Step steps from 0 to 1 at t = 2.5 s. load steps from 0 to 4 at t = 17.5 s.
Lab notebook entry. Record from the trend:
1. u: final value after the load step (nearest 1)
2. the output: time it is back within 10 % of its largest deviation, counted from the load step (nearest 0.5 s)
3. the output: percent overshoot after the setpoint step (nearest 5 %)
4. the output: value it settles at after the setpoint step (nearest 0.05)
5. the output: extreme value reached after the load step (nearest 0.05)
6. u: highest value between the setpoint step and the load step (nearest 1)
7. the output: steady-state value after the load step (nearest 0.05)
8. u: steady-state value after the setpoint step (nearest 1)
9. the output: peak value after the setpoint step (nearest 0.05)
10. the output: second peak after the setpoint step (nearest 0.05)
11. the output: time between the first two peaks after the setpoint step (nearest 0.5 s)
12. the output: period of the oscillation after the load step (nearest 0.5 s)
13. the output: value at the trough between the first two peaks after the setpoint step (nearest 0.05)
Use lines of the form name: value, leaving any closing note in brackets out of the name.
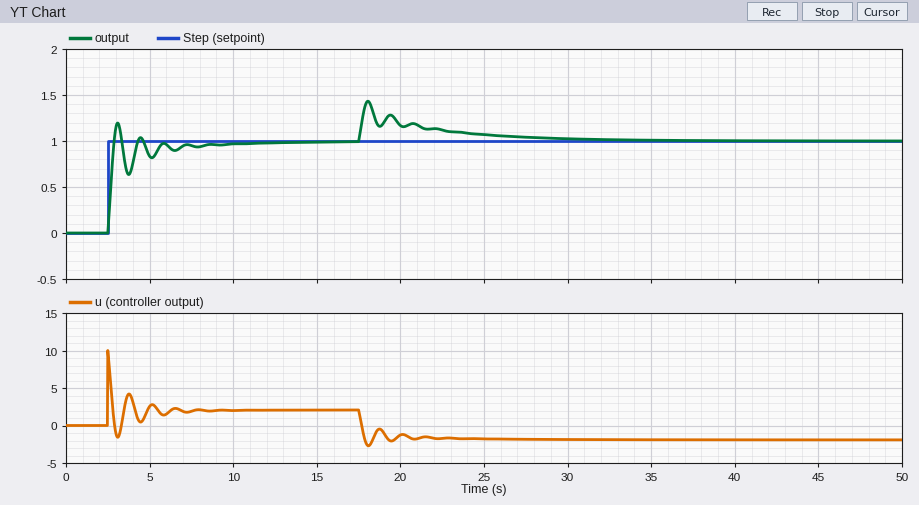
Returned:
u: final value after the load step: -2
the output: time it is back within 10 % of its largest deviation, counted from the load step: 9.5 s
the output: percent overshoot after the setpoint step: 20 %
the output: value it settles at after the setpoint step: 1.00
the output: extreme value reached after the load step: 1.45
u: highest value between the setpoint step and the load step: 10
the output: steady-state value after the load step: 1.00
u: steady-state value after the setpoint step: 2
the output: peak value after the setpoint step: 1.20
the output: second peak after the setpoint step: 1.05
the output: time between the first two peaks after the setpoint step: 1.5 s
the output: period of the oscillation after the load step: 1.5 s
the output: value at the trough between the first two peaks after the setpoint step: 0.65
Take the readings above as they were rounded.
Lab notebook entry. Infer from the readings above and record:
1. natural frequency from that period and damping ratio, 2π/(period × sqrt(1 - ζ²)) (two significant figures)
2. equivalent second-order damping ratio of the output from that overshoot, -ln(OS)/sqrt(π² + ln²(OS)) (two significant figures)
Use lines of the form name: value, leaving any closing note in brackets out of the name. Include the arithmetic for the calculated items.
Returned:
natural frequency from that period and damping ratio, 2π/(period × sqrt(1 - ζ²)): 2π / (1.5 × sqrt(1 - 0.46²)) = 4.7 rad/s
equivalent second-order damping ratio of the output from that overshoot, -ln(OS)/sqrt(π² + ln²(OS)): ln(0.2) = -1.609; 1.609 / sqrt(9.870 + 2.590) = 0.46
